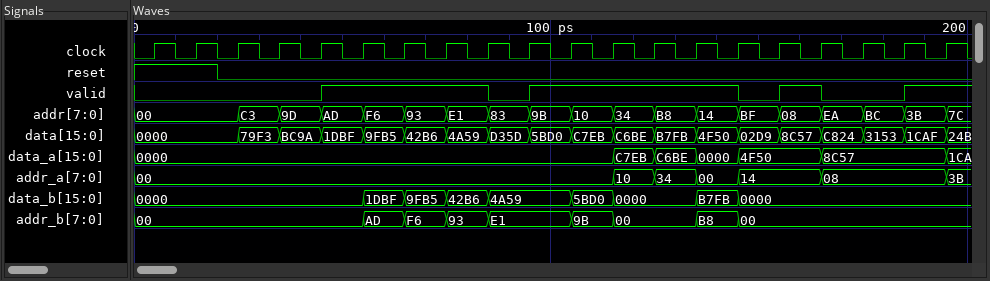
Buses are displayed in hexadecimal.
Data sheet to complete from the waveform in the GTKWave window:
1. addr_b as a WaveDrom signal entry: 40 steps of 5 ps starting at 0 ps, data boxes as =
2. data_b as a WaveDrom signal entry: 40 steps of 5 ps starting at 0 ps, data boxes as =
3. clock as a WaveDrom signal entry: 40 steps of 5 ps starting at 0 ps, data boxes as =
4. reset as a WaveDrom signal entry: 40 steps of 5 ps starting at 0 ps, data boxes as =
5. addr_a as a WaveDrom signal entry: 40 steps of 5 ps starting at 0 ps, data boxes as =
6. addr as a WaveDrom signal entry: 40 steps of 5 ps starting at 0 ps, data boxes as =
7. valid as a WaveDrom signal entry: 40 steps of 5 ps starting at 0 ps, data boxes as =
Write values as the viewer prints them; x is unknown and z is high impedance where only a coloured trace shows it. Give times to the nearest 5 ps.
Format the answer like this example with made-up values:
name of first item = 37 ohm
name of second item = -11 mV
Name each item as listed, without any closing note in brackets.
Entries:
addr_b as a WaveDrom signal entry: 40 steps of 5 ps starting at 0 ps, data boxes as = = {name: 'addr_b', wave: '=..........=.=.=.=...=.=...=.=..........', data: '00 AD F6 93 E1 9B 00 B8 00'}
data_b as a WaveDrom signal entry: 40 steps of 5 ps starting at 0 ps, data boxes as = = {name: 'data_b', wave: '=..........=.=.=.=...=.=...=.=..........', data: '0000 1DBF 9FB5 42B6 4A59 5BD0 0000 B7FB 0000'}
clock as a WaveDrom signal entry: 40 steps of 5 ps starting at 0 ps, data boxes as = = {name: 'clock', wave: '0101010101010101010101010101010101010101'}
reset as a WaveDrom signal entry: 40 steps of 5 ps starting at 0 ps, data boxes as = = {name: 'reset', wave: '1...0...................................'}
addr_a as a WaveDrom signal entry: 40 steps of 5 ps starting at 0 ps, data boxes as = = {name: 'addr_a', wave: '=......................=.=.=.=...=.....=', data: '00 10 34 00 14 08 3B'}
addr as a WaveDrom signal entry: 40 steps of 5 ps starting at 0 ps, data boxes as = = {name: 'addr', wave: '=....=.=.=.=.=.=.=.=.=.=.=.=.=.=.=.=.=.=', data: '00 C3 9D AD F6 93 E1 83 9B 10 34 B8 14 BF 08 EA BC 3B 7C'}
valid as a WaveDrom signal entry: 40 steps of 5 ps starting at 0 ps, data boxes as = = {name: 'valid', wave: '0........1.......0.1.........0.1.0...1..'}
